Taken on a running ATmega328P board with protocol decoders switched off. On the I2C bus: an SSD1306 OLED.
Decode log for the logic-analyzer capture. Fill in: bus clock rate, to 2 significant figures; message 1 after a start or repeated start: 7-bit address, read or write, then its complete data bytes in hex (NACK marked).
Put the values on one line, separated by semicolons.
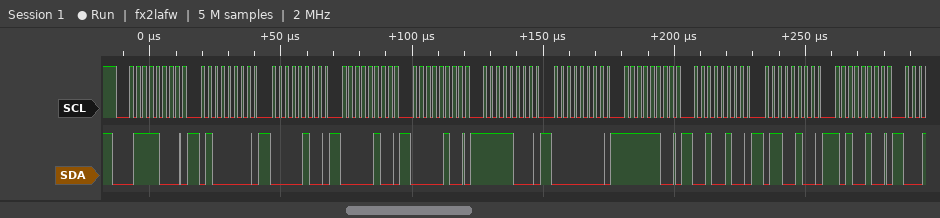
400 kHz; 0x3C write: 40 04 04 04 F8 00 FC 24 64 A4
